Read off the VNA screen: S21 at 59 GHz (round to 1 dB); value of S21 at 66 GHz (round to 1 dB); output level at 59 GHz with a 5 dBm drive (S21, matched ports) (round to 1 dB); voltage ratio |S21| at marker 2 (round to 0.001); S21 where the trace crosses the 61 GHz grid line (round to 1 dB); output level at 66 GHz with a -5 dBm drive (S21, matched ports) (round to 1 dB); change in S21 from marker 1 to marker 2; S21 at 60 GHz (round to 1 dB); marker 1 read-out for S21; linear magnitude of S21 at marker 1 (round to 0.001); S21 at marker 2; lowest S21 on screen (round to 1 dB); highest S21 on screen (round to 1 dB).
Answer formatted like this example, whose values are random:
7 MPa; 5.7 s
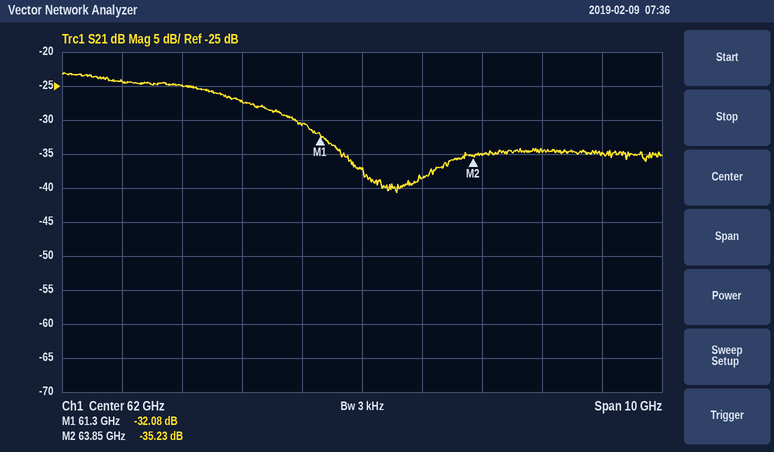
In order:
-25 dB; -35 dB; -20 dBm; 0.017; -31 dB; -40 dBm; -3.15 dB; -27 dB; -32.08 dB; 0.025; -35.23 dB; -41 dB; -23 dB
